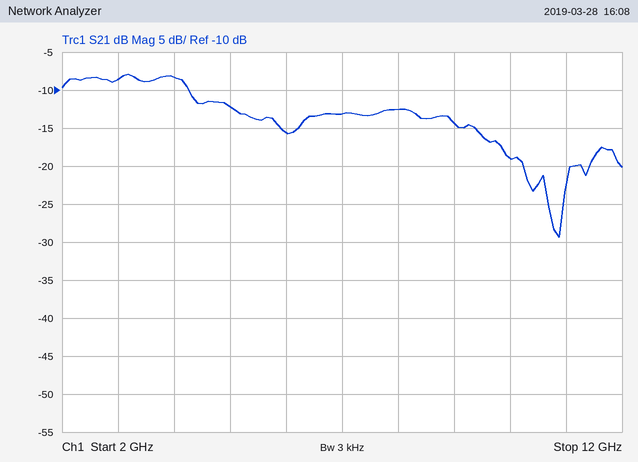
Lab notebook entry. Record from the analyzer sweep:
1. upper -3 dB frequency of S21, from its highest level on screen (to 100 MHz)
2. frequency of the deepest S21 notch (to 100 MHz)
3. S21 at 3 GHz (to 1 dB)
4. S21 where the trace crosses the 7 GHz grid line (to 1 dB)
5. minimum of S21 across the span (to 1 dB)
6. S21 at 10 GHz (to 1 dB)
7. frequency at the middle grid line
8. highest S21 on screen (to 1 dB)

4.3 GHz
10.9 GHz
-9 dB
-13 dB
-29 dB
-19 dB
7 GHz
-8 dB
